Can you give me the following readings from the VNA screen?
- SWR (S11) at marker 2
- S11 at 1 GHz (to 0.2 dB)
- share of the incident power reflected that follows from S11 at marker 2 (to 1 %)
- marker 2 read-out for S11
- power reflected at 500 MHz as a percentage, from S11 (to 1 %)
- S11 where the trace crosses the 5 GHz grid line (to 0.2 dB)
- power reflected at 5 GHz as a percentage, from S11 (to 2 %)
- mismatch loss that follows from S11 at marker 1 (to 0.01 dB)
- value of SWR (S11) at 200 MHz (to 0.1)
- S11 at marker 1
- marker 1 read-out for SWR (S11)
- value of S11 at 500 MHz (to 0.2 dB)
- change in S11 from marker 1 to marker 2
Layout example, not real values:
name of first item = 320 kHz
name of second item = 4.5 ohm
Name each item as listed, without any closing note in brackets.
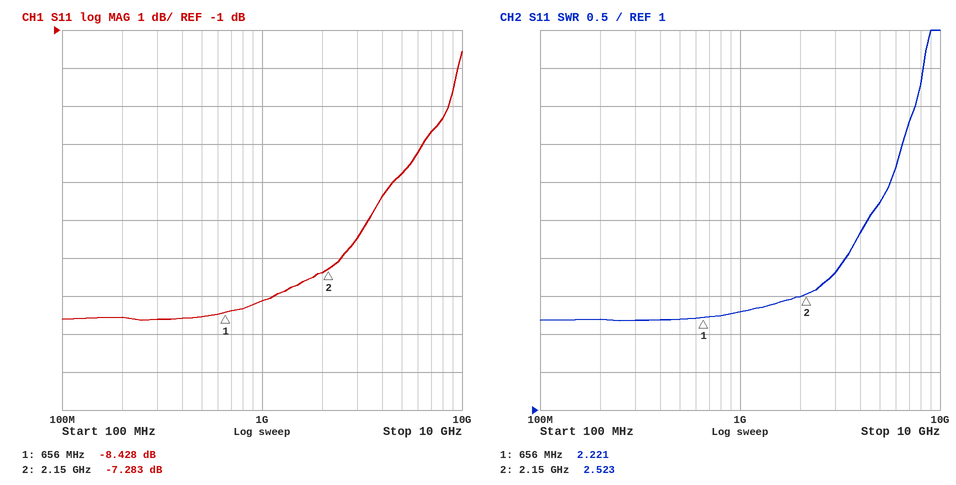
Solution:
SWR (S11) at marker 2 = 2.523
S11 at 1 GHz = -8.2 dB
share of the incident power reflected that follows from S11 at marker 2 = 19 %
marker 2 read-out for S11 = -7.283 dB
power reflected at 500 MHz as a percentage, from S11 = 14 %
S11 where the trace crosses the 5 GHz grid line = -4.8 dB
power reflected at 5 GHz as a percentage, from S11 = 34 %
mismatch loss that follows from S11 at marker 1 = 0.67 dB
value of SWR (S11) at 200 MHz = 2.2
S11 at marker 1 = -8.428 dB
marker 1 read-out for SWR = 2.221
value of S11 at 500 MHz = -8.6 dB
change in S11 from marker 1 to marker 2 = 1.145 dB
